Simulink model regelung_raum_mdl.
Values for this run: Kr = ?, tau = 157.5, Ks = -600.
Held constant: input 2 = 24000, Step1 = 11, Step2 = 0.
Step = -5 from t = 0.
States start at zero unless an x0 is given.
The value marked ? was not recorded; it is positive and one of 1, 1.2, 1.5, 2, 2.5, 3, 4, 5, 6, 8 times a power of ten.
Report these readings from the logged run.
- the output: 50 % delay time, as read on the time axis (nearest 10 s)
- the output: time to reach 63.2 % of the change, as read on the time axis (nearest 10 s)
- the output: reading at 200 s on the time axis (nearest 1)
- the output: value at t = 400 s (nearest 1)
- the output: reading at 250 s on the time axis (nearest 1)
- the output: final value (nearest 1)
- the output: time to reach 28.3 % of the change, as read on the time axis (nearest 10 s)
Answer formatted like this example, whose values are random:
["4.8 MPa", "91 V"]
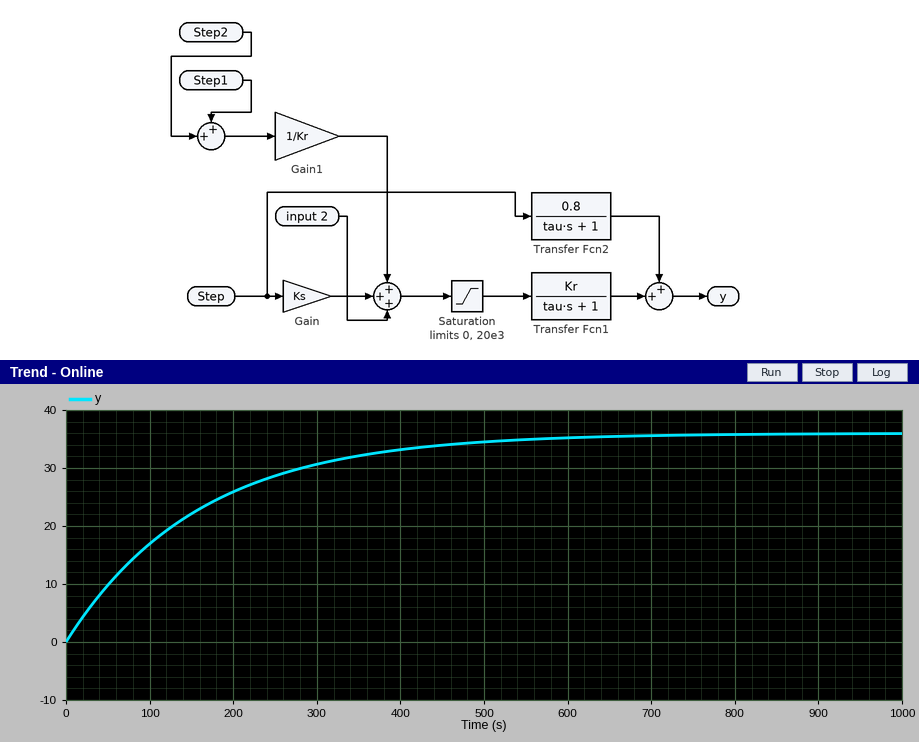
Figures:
["110 s", "160 s", "26", "33", "29", "36", "50 s"]
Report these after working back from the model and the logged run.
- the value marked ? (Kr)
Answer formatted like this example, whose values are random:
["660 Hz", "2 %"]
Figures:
["0.002"]
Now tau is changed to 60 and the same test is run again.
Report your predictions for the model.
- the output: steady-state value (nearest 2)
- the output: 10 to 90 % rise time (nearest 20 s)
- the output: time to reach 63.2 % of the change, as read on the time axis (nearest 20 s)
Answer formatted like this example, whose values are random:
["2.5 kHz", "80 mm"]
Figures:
["36", "140 s", "60 s"]
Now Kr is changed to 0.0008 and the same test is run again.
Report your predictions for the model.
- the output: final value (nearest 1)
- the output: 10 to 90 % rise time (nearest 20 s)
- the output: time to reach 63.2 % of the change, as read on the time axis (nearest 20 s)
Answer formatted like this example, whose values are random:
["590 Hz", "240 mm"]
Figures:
["12", "340 s", "160 s"]
